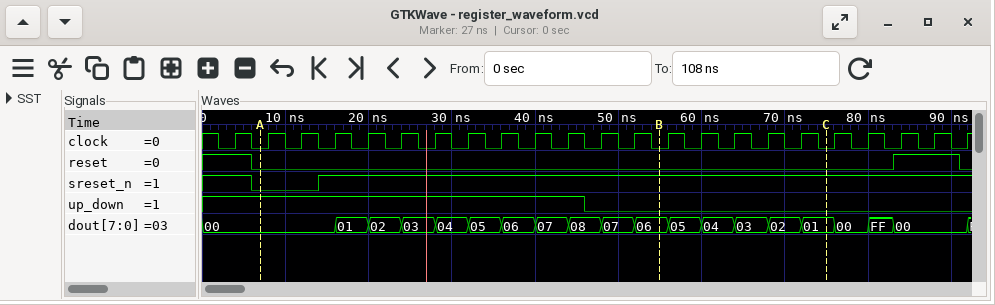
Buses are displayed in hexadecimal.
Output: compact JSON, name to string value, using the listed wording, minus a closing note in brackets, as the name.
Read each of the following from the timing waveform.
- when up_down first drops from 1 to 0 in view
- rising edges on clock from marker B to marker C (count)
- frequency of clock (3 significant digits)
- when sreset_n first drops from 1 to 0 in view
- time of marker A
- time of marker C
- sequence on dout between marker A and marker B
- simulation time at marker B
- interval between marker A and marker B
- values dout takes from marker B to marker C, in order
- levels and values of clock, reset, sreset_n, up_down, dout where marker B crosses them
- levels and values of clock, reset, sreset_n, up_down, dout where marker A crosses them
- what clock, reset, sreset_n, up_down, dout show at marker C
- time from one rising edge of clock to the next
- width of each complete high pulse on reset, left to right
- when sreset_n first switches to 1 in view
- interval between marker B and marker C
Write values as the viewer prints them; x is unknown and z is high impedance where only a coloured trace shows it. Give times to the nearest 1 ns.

{"when up_down first drops from 1 to 0 in view": "46 ns", "rising edges on clock from marker B to marker C": "5", "frequency of clock": "250 MHz", "when sreset_n first drops from 1 to 0 in view": "6 ns", "time of marker A": "7 ns", "time of marker C": "75 ns", "sequence on dout between marker A and marker B": "00, 01, 02, 03, 04, 05, 06, 07, 08, 07, 06", "simulation time at marker B": "55 ns", "interval between marker A and marker B": "48 ns", "values dout takes from marker B to marker C, in order": "06, 05, 04, 03, 02, 01", "levels and values of clock, reset, sreset_n, up_down, dout where marker B crosses them": "clock=0, reset=0, sreset_n=1, up_down=0, dout=06", "levels and values of clock, reset, sreset_n, up_down, dout where marker A crosses them": "clock=0, reset=0, sreset_n=0, up_down=1, dout=00", "what clock, reset, sreset_n, up_down, dout show at marker C": "clock=0, reset=0, sreset_n=1, up_down=0, dout=01", "time from one rising edge of clock to the next": "4 ns", "width of each complete high pulse on reset, left to right": "8 ns", "when sreset_n first switches to 1 in view": "14 ns", "interval between marker B and marker C": "20 ns"}
